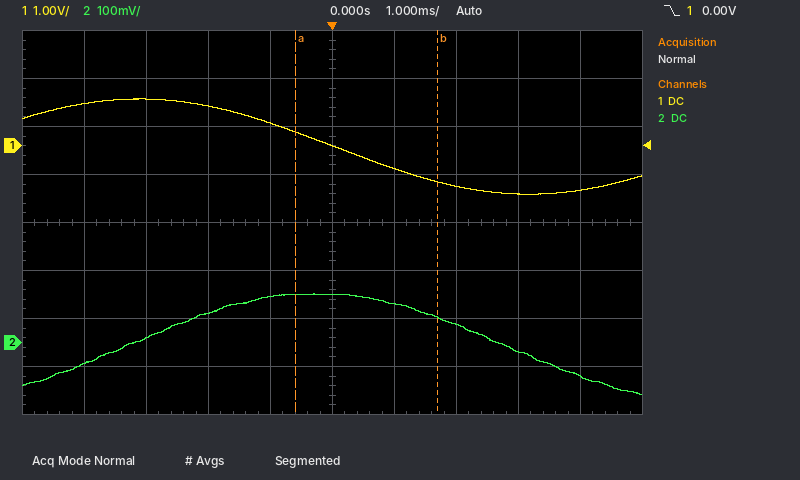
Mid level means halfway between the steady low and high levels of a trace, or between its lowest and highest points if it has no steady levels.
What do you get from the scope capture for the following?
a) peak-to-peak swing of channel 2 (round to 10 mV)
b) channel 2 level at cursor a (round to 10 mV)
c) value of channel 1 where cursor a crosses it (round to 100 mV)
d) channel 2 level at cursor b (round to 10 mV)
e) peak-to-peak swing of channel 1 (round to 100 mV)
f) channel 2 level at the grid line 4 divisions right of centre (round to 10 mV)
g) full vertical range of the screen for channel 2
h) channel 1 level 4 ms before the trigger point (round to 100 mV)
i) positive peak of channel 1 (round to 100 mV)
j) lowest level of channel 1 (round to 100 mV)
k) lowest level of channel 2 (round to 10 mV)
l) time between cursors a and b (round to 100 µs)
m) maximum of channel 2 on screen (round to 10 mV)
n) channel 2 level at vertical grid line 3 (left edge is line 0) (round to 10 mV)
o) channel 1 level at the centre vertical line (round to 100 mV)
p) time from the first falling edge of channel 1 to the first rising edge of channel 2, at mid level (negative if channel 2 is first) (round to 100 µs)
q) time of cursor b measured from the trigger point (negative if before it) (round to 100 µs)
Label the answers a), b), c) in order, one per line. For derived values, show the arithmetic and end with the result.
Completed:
a) 100 mV − (-110 mV) = 210 mV
b) 100 mV
c) 300 mV
d) 50 mV
e) 1.0 V − (-1.0 V) = 2.0 V
f) -70 mV
g) 800 mV
h) 900 mV
i) 1.0 V
j) -1.0 V
k) -110 mV
l) 2.3 ms
m) 100 mV
n) 60 mV
o) 0.0 V
p) -3.3 ms
q) +1.7 ms
